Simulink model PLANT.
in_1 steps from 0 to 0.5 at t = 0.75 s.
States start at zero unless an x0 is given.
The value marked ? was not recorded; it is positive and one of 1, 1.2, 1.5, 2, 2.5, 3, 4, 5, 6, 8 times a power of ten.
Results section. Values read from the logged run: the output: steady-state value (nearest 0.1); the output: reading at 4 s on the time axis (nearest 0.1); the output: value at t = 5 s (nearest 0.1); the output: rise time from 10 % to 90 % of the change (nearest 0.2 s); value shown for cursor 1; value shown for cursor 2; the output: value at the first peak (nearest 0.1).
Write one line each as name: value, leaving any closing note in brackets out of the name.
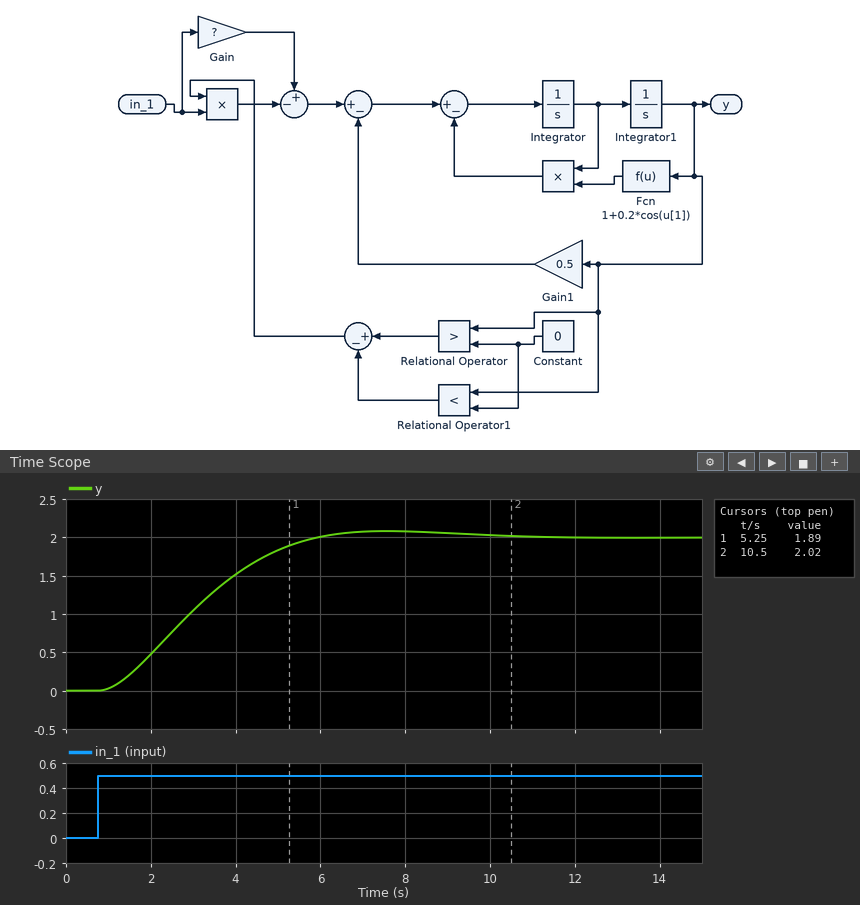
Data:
the output: steady-state value: 2.0
the output: reading at 4 s on the time axis: 1.5
the output: value at t = 5 s: 1.8
the output: rise time from 10 % to 90 % of the change: 3.4 s
value shown for cursor 1: 1.89
value shown for cursor 2: 2.02
the output: value at the first peak: 2.1
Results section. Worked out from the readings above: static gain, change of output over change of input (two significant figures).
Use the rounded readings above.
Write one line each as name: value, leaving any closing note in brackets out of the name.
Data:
static gain, change of output over change of input: 4.0
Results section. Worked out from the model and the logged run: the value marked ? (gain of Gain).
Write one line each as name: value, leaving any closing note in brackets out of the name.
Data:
the value marked ?: 3
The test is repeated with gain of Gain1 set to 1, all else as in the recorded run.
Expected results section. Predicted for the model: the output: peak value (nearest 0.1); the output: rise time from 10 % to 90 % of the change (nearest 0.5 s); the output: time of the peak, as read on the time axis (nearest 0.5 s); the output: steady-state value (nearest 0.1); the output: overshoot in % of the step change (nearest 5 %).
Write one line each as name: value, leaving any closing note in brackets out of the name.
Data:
the output: peak value: 1.1
the output: rise time from 10 % to 90 % of the change: 2.0 s
the output: time of the peak, as read on the time axis: 4.5 s
the output: steady-state value: 1.0
the output: overshoot in % of the step change: 10 %
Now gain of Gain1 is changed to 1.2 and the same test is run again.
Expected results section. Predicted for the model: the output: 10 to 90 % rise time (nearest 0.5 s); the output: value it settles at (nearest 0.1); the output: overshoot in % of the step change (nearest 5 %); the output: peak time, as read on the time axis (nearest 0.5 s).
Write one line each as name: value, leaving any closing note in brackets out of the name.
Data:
the output: 10 to 90 % rise time: 1.5 s
the output: value it settles at: 0.8
the output: overshoot in % of the step change: 15 %
the output: peak time, as read on the time axis: 4.0 s
